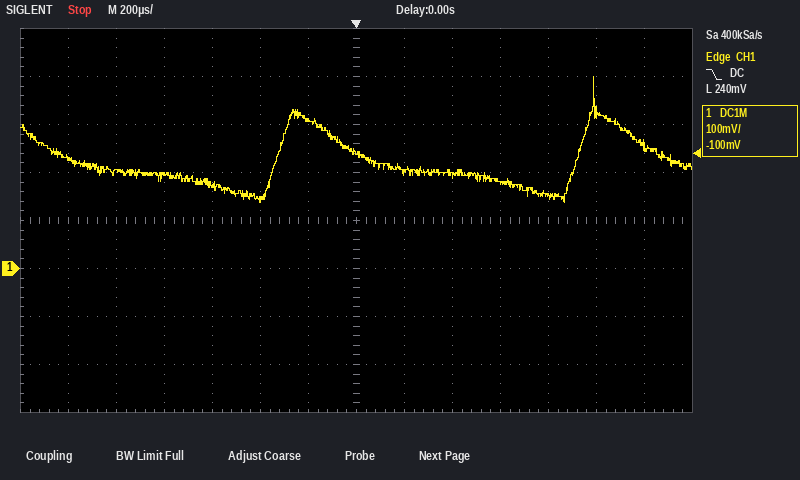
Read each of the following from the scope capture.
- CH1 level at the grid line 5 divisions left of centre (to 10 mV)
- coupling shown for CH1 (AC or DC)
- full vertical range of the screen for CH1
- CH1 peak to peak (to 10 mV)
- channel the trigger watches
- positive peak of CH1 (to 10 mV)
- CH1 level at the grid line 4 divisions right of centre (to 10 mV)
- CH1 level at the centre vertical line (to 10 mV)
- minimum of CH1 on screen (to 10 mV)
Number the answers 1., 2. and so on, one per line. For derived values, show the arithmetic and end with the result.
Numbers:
1. 200 mV
2. DC
3. 800 mV
4. 400 mV − (140 mV) = 260 mV
5. CH1
6. 400 mV
7. 150 mV
8. 240 mV
9. 140 mV
